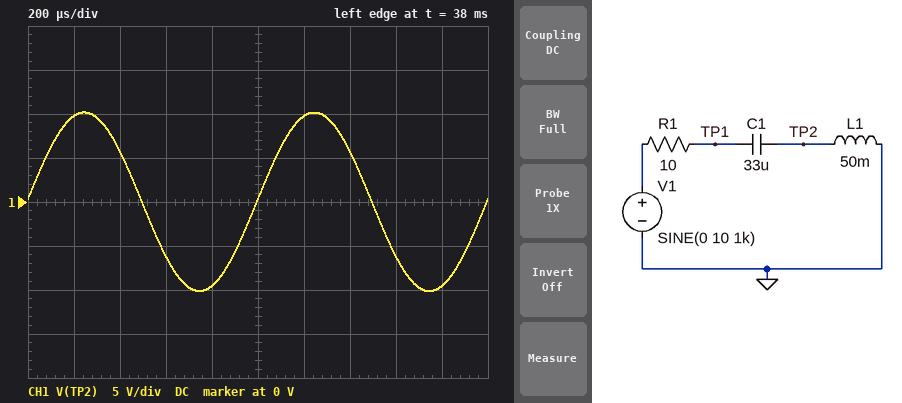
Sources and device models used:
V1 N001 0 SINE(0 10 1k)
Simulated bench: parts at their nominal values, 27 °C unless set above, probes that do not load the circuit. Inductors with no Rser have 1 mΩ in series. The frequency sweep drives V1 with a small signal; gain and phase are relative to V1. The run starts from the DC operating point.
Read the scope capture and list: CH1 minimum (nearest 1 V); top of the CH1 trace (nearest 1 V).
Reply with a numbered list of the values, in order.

1. -10 V
2. 10 V
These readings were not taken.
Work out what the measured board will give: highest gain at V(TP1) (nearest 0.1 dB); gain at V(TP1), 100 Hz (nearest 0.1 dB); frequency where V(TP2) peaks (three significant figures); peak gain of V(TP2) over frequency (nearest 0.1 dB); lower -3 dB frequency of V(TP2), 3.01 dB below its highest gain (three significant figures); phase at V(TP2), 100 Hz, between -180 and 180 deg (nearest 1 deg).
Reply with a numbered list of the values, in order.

1. 0 dB
2. -1.3 dB
3. 126 Hz
4. 11.9 dB
5. 112 Hz
6. 149 deg
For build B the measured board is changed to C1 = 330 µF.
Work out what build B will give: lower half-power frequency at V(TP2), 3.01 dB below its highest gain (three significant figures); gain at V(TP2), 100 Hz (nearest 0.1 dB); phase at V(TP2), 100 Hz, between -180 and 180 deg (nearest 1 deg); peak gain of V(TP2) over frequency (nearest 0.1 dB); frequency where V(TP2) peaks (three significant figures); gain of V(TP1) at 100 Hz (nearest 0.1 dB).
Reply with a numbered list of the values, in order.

1. 33.0 Hz
2. 0.9 dB
3. 21 deg
4. 2.6 dB
5. 47.9 Hz
6. -0.6 dB
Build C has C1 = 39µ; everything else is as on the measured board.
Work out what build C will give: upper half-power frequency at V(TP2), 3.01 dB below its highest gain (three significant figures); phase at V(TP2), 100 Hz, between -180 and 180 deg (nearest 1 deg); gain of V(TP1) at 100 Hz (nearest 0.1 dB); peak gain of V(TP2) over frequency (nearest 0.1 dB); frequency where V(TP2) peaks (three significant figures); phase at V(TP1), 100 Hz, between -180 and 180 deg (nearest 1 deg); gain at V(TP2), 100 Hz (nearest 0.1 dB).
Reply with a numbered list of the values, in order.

1. 138 Hz
2. 133 deg
3. -3.3 dB
4. 11.2 dB
5. 116 Hz
6. -47 deg
7. 7.2 dB
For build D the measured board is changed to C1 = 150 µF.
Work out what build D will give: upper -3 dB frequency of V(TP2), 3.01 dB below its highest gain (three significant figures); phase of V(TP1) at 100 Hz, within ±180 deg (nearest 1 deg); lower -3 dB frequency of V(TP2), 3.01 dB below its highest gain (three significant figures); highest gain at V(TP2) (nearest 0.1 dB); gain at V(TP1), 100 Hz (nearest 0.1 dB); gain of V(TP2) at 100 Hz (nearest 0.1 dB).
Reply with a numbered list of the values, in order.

1. 102 Hz
2. 26 deg
3. 49.5 Hz
4. 5.6 dB
5. -0.9 dB
6. 2.7 dB
